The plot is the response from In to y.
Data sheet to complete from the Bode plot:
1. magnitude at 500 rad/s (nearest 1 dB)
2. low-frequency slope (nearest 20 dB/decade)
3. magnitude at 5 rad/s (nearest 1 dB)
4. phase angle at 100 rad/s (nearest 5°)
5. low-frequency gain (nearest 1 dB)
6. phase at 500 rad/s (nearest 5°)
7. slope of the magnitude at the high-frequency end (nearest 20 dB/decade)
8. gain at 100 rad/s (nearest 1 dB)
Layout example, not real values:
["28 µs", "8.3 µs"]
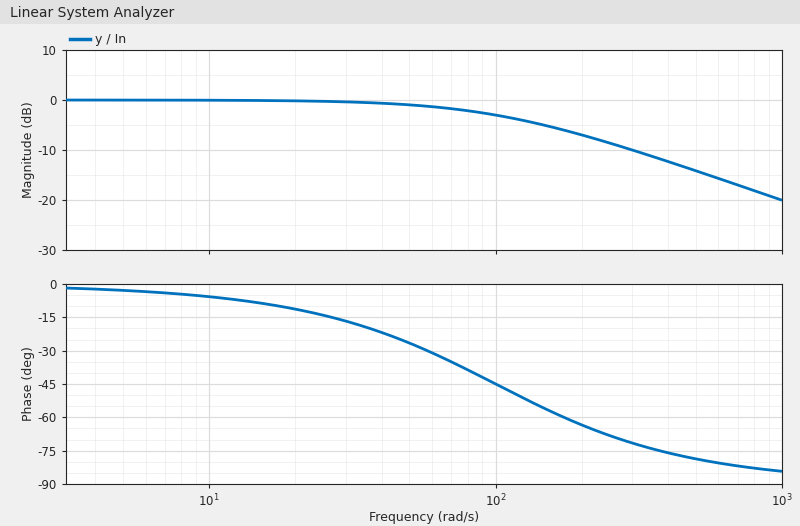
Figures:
["-14 dB", "0 dB/decade", "0 dB", "-45°", "0 dB", "-80°", "-20 dB/decade", "-3 dB"]
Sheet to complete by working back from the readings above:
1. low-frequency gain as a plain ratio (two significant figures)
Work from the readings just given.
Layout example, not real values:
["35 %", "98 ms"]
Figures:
["1.0"]
